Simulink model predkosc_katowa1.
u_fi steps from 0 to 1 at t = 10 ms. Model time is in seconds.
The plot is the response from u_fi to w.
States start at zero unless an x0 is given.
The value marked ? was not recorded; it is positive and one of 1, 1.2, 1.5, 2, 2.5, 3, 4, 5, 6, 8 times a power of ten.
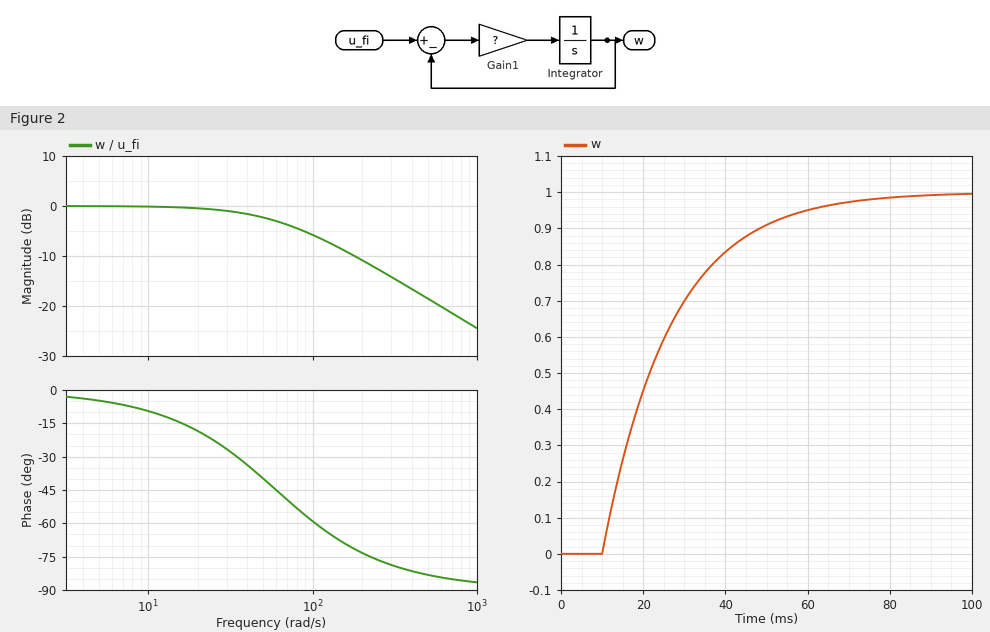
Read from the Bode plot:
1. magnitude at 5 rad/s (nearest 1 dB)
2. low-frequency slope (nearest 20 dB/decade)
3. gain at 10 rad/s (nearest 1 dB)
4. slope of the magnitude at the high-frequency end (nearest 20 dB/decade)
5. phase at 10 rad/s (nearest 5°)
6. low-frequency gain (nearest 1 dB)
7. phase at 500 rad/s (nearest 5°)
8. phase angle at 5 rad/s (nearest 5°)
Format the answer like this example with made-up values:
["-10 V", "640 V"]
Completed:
["0 dB", "0 dB/decade", "0 dB", "-20 dB/decade", "-10°", "0 dB", "-85°", "-5°"]
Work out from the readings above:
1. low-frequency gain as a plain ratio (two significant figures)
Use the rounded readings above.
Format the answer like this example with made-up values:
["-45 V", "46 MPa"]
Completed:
["1.0"]
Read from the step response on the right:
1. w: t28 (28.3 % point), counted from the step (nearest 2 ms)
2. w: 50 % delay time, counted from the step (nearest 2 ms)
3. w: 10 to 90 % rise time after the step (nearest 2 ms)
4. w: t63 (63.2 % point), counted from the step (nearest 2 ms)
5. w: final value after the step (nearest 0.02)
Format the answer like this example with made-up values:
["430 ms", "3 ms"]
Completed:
["6 ms", "12 ms", "36 ms", "16 ms", "1.00"]
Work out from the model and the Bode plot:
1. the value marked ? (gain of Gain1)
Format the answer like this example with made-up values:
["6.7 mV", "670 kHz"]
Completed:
["60"]
